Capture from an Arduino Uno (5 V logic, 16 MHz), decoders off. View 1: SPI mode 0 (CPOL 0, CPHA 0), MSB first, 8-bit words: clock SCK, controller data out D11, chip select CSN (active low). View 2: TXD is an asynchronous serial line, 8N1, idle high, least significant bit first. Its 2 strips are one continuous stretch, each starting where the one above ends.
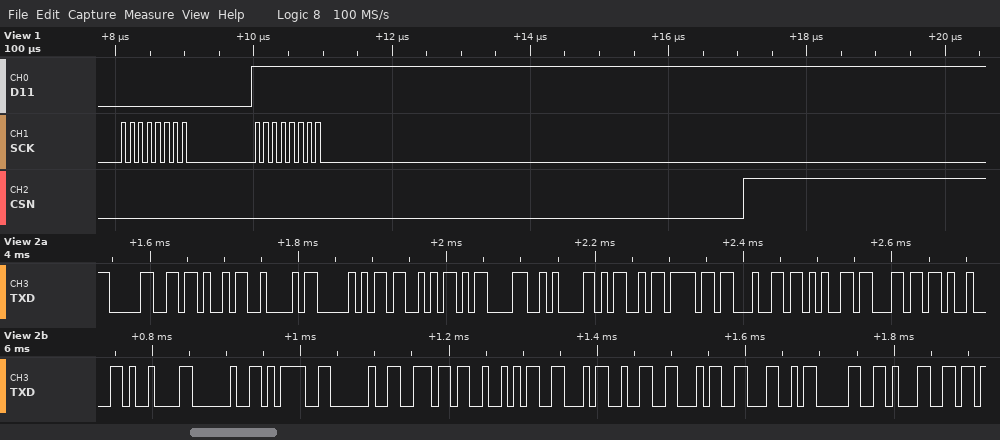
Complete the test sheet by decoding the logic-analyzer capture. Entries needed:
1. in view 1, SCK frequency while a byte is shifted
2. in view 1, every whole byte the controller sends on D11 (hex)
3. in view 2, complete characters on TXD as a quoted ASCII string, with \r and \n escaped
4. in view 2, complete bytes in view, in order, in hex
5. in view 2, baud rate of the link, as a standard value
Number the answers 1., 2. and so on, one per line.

1. 8 MHz
2. 00 FF
3. "0KBPS\r\nModel\t\t = nRF24L01"
4. 30 4B 42 50 53 0D 0A 4D 6F 64 65 6C 09 09 20 3D 20 6E 52 46 32 34 4C 30 31
5. 115200 baud
